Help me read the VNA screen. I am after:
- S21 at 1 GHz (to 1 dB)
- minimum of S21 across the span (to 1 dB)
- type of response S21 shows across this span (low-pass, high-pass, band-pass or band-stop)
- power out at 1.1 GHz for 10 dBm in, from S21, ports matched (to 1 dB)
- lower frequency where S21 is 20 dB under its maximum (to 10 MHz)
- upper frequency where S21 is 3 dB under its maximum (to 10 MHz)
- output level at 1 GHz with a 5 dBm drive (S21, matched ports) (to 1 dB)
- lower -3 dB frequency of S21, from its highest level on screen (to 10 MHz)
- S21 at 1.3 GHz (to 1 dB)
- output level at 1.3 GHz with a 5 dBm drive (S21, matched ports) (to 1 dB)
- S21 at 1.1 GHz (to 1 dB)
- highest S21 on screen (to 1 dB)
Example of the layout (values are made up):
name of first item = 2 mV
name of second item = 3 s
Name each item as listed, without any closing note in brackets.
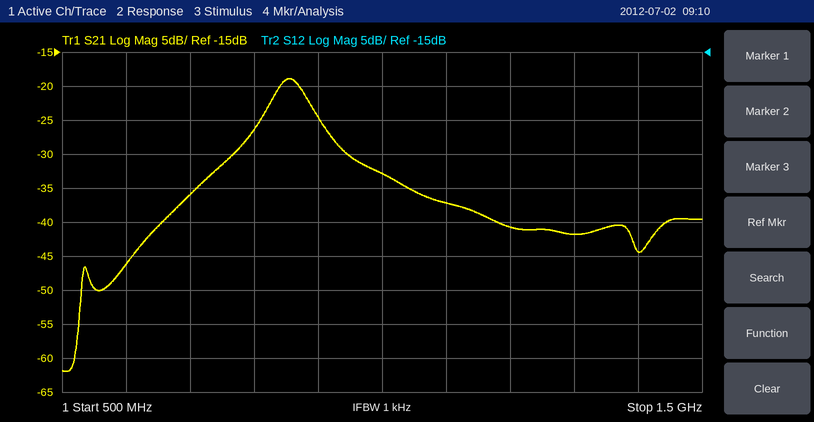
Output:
S21 at 1 GHz = -33 dB
minimum of S21 across the span = -62 dB
type of response S21 shows across this span = band-pass
power out at 1.1 GHz for 10 dBm in, from S21, ports matched = -27 dBm
lower frequency where S21 is 20 dB under its maximum = 670 MHz
upper frequency where S21 is 3 dB under its maximum = 880 MHz
output level at 1 GHz with a 5 dBm drive (S21, matched ports) = -28 dBm
lower -3 dB frequency of S21, from its highest level on screen = 830 MHz
S21 at 1.3 GHz = -42 dB
output level at 1.3 GHz with a 5 dBm drive (S21, matched ports) = -37 dBm
S21 at 1.1 GHz = -37 dB
highest S21 on screen = -19 dB
